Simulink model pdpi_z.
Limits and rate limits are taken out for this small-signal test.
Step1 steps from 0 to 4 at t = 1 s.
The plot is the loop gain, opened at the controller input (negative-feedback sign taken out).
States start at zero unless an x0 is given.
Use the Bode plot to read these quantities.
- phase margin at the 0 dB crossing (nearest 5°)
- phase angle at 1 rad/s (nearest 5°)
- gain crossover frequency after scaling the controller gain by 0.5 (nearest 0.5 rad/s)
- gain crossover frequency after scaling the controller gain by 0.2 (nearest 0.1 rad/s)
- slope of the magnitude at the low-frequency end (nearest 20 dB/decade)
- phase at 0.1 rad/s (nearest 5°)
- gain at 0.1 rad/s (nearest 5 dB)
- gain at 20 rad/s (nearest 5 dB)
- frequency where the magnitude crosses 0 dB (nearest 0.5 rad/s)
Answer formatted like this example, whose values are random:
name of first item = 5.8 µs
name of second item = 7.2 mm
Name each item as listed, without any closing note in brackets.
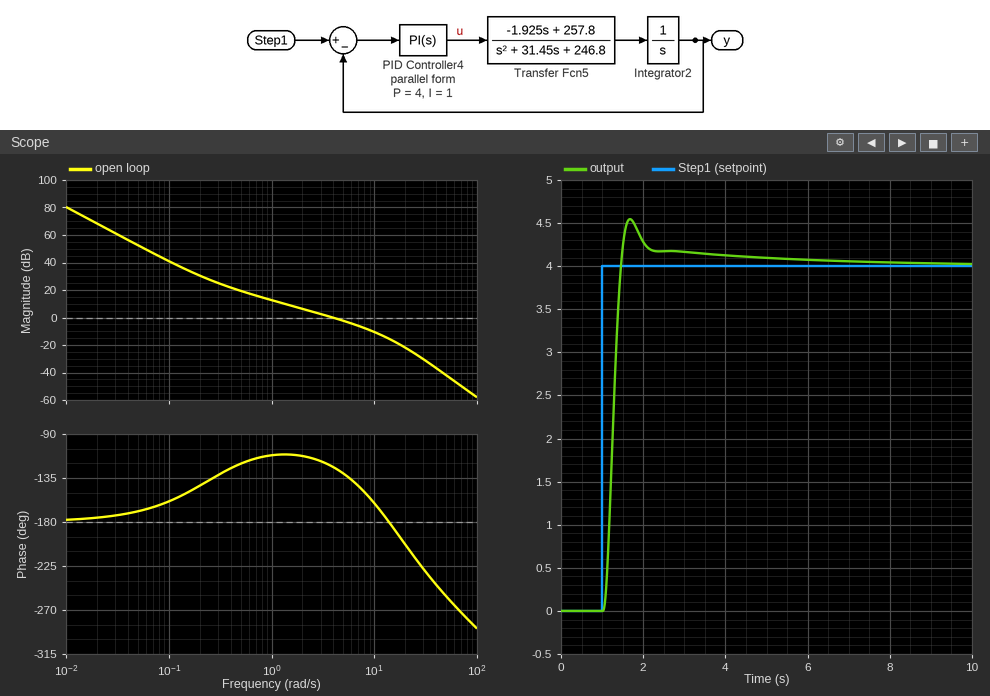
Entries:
phase margin at the 0 dB crossing = 55°
phase angle at 1 rad/s = -110°
gain crossover frequency after scaling the controller gain by 0.5 = 2.0 rad/s
gain crossover frequency after scaling the controller gain by 0.2 = 0.9 rad/s
slope of the magnitude at the low-frequency end = -40 dB/decade
phase at 0.1 rad/s = -160°
gain at 0.1 rad/s = 40 dB
gain at 20 rad/s = -20 dB
frequency where the magnitude crosses 0 dB = 4.0 rad/s
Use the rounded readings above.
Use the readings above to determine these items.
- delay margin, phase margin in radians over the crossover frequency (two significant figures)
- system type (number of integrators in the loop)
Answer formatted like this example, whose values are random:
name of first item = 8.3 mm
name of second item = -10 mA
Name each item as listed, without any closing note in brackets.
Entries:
delay margin, phase margin in radians over the crossover frequency = 0.24 s
system type = 2
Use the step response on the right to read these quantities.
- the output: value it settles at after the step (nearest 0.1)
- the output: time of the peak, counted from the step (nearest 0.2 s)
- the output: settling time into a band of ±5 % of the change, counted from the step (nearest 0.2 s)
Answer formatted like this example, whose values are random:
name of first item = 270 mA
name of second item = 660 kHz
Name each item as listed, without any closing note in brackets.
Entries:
the output: value it settles at after the step = 4.0
the output: time of the peak, counted from the step = 0.6 s
the output: settling time into a band of ±5 % of the change, counted from the step = 1.2 s
